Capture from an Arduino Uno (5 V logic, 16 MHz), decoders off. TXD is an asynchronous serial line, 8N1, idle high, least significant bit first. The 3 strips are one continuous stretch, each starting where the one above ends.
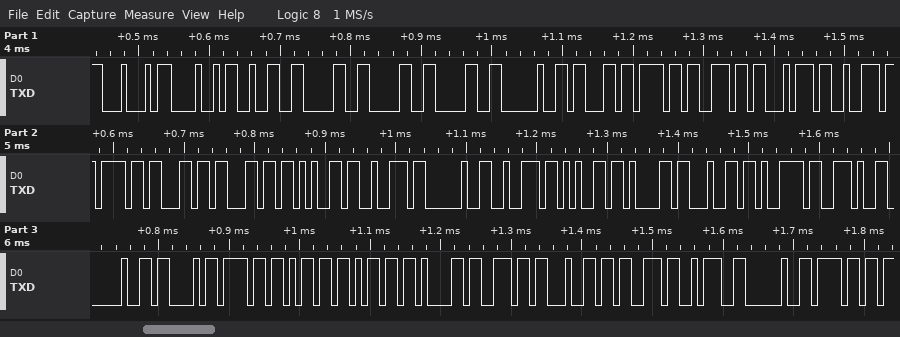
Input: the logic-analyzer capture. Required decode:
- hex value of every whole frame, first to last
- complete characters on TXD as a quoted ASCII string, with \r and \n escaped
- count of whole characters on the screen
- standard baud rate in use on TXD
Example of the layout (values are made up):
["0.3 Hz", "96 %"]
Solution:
["0x44 0x48 0x32 0x30 0x30 0x30 0x20 0x63 0x6F 0x6E 0x74 0x72 0x6F 0x6C 0x6C 0x65 0x72 0x20 0x72 0x65 0x61 0x64 0x79 0x2E 0x20 0x43 0x6F 0x6D 0x6D 0x61 0x6E 0x64 0x73 0x3A 0x20 0x6F", "\"DH2000 controller ready. Commands: o\"", "36", "115200 baud"]
